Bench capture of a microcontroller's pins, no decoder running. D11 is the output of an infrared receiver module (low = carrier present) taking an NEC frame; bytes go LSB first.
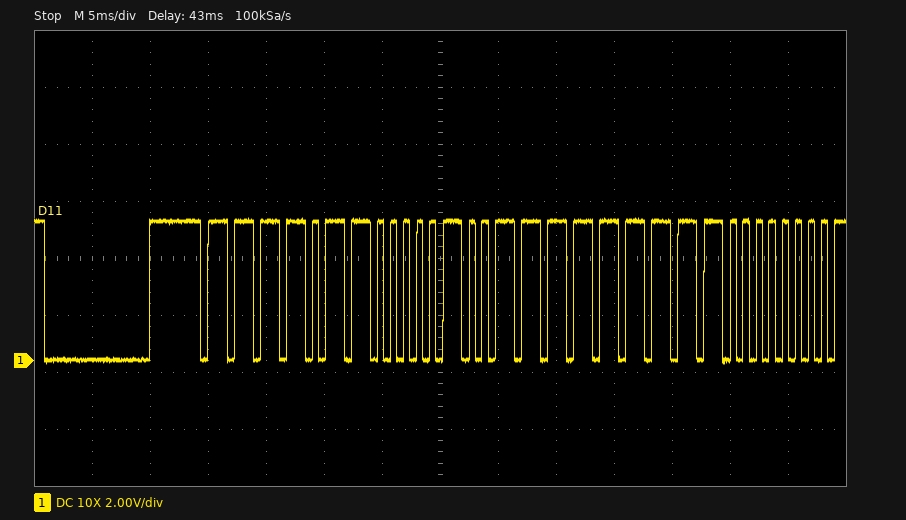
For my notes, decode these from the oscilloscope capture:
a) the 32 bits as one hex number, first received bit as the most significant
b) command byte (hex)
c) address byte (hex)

0xF609FF00
0xFF
0x6F
